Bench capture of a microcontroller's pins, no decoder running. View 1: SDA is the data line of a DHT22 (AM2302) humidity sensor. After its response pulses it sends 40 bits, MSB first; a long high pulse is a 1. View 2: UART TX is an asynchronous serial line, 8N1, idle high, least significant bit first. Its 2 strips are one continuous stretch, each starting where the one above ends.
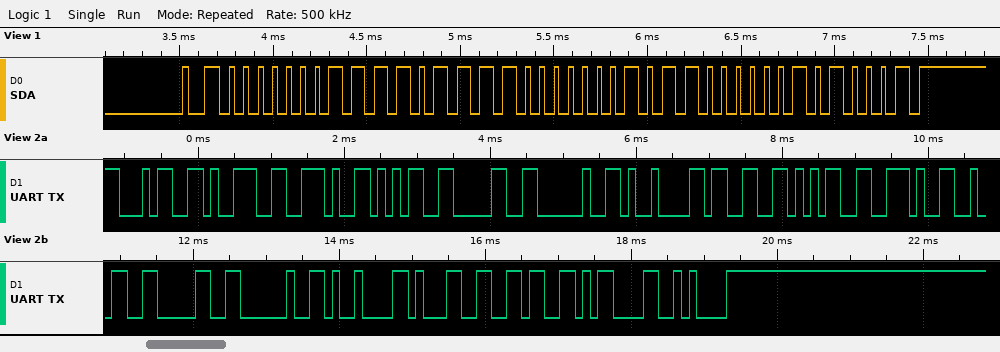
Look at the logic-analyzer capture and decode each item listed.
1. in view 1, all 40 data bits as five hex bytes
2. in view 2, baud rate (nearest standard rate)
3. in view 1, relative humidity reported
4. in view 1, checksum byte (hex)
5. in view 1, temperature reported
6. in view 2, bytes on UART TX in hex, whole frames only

01 EF 01 60 51
9600 baud
49.5 %
0x51
35.2 °C
34 39 2E 35 30 20 09 33 35 2E 32 30 20 09 31 36 0D 0A
